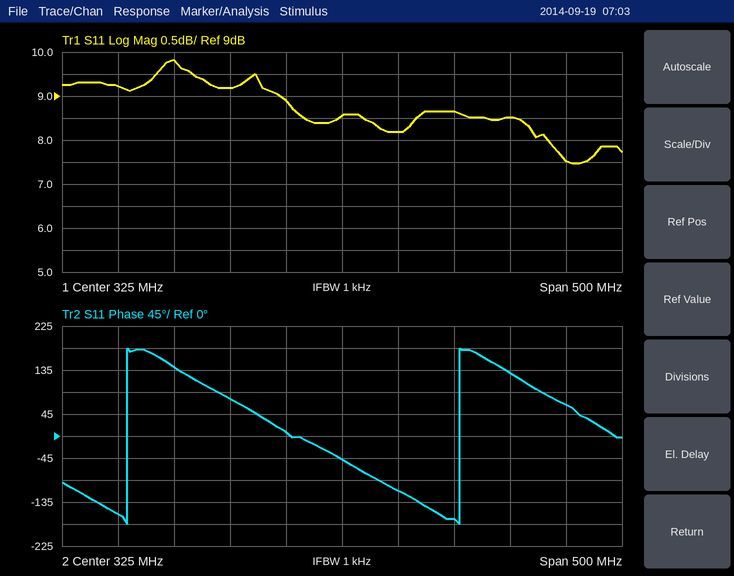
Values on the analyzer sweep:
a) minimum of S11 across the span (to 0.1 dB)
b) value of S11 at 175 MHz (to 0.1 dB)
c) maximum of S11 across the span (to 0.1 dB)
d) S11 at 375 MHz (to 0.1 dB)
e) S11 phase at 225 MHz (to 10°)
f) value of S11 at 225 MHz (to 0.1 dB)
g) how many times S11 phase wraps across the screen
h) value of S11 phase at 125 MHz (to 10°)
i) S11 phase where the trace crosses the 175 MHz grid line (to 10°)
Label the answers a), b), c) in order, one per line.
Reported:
a) 7.5 dB
b) 9.8 dB
c) 9.8 dB
d) 8.2 dB
e) 80°
f) 9.2 dB
g) 2
h) -160°
i) 140°
